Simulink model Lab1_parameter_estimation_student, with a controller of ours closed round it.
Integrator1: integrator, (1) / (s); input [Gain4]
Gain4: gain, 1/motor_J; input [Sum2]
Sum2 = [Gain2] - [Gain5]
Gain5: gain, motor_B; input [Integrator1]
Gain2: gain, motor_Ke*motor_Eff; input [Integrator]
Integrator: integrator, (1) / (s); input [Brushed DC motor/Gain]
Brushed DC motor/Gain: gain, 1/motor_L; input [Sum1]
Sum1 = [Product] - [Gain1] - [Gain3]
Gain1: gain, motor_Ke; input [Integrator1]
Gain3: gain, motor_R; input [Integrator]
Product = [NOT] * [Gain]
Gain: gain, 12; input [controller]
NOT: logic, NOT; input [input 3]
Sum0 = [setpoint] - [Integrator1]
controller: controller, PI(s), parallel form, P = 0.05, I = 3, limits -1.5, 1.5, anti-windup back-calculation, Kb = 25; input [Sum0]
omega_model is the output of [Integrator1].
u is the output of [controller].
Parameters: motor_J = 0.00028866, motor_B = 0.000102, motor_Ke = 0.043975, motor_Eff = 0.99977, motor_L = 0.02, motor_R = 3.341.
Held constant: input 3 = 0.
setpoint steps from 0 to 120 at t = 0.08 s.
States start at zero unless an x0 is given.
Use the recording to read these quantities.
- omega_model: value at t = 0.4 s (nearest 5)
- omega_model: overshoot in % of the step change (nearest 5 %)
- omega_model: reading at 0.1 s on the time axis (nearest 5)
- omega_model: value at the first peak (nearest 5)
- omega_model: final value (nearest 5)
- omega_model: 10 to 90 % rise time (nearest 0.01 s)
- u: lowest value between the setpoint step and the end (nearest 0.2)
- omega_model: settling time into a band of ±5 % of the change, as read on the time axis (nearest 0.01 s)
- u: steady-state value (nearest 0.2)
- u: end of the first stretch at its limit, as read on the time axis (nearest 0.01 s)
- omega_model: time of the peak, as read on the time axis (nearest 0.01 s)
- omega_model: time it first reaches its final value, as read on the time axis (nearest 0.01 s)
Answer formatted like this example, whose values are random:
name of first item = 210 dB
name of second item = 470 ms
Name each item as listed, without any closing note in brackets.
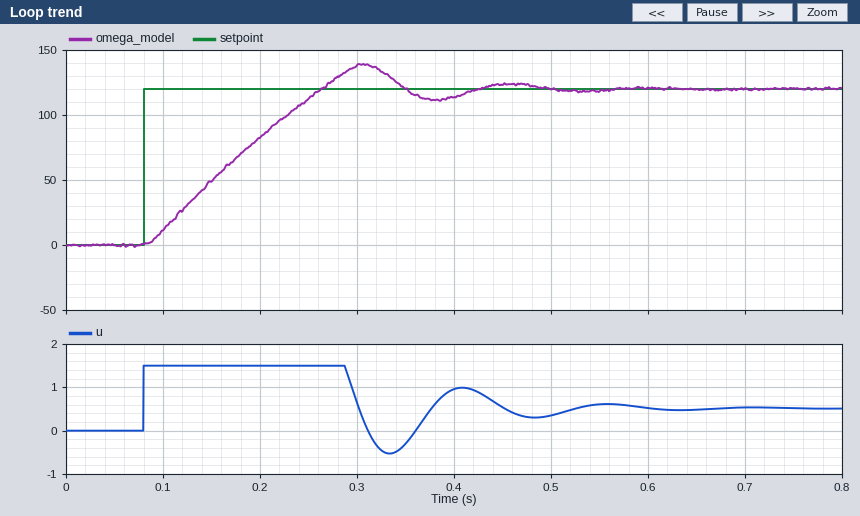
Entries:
omega_model: value at t = 0.4 s = 115
omega_model: overshoot in % of the step change = 15 %
omega_model: reading at 0.1 s on the time axis = 10
omega_model: value at the first peak = 140
omega_model: final value = 120
omega_model: 10 to 90 % rise time = 0.14 s
u: lowest value between the setpoint step and the end = -0.6
omega_model: settling time into a band of ±5 % of the change, as read on the time axis = 0.40 s
u: steady-state value = 0.6
u: end of the first stretch at its limit, as read on the time axis = 0.29 s
omega_model: time of the peak, as read on the time axis = 0.31 s
omega_model: time it first reaches its final value, as read on the time axis = 0.26 s
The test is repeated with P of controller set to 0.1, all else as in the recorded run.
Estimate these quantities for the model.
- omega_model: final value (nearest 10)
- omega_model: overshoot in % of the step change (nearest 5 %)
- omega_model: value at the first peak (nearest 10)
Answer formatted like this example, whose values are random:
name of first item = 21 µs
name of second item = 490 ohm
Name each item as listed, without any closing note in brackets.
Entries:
omega_model: final value = 120
omega_model: overshoot in % of the step change = 10 %
omega_model: value at the first peak = 130
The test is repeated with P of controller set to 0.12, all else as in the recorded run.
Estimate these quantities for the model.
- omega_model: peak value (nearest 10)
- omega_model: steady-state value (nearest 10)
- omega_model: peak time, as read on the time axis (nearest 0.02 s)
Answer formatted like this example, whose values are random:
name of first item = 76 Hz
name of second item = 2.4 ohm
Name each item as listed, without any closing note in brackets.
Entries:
omega_model: peak value = 130
omega_model: steady-state value = 120
omega_model: peak time, as read on the time axis = 0.28 s
